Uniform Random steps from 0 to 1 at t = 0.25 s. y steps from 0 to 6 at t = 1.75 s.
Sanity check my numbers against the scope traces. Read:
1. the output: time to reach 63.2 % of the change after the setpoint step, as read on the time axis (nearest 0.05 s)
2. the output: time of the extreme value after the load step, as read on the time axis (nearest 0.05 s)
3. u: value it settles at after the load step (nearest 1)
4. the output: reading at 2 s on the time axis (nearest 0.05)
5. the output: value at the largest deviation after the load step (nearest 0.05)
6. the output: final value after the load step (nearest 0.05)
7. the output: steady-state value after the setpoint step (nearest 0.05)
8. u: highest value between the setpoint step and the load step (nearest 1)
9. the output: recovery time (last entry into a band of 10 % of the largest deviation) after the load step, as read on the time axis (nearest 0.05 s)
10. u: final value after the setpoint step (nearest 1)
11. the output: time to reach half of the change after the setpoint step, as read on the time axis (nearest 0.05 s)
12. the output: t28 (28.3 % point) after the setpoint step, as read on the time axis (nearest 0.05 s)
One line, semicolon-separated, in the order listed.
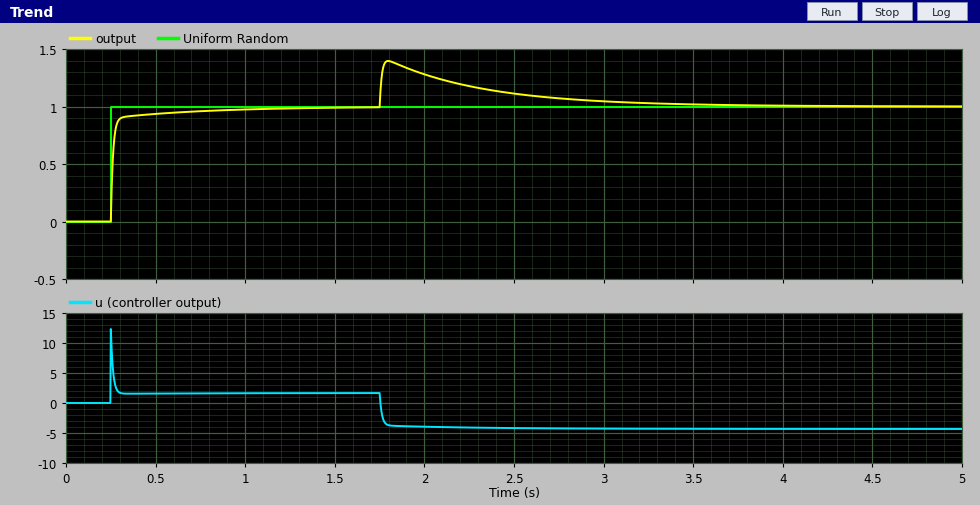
0.25 s; 1.80 s; -4; 1.30; 1.40; 1.00; 1.00; 12; 3.05 s; 2; 0.25 s; 0.25 s
